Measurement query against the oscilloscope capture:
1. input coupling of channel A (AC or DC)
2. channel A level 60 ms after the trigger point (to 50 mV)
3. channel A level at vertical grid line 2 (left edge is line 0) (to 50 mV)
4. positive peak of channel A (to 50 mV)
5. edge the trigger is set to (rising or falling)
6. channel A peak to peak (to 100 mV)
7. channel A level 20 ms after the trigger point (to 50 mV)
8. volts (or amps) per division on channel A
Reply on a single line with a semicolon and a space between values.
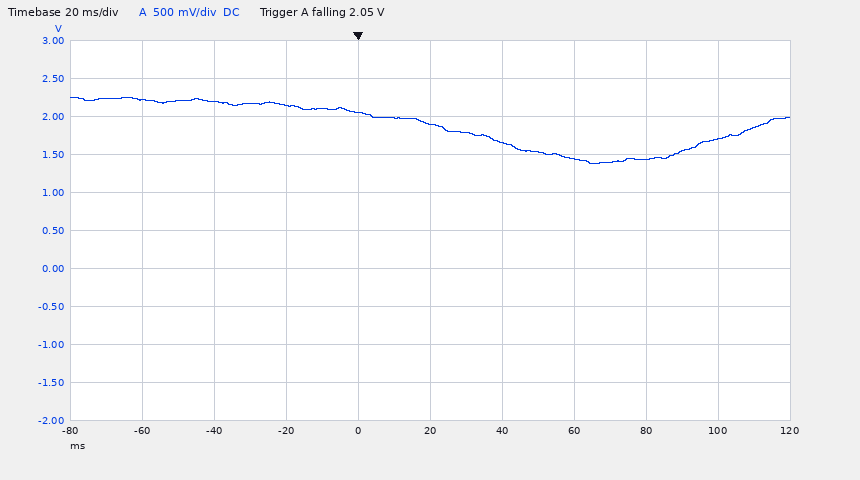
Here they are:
DC; 1.45 V; 2.20 V; 2.25 V; falling; 900 mV; 1.90 V; 500 mV
